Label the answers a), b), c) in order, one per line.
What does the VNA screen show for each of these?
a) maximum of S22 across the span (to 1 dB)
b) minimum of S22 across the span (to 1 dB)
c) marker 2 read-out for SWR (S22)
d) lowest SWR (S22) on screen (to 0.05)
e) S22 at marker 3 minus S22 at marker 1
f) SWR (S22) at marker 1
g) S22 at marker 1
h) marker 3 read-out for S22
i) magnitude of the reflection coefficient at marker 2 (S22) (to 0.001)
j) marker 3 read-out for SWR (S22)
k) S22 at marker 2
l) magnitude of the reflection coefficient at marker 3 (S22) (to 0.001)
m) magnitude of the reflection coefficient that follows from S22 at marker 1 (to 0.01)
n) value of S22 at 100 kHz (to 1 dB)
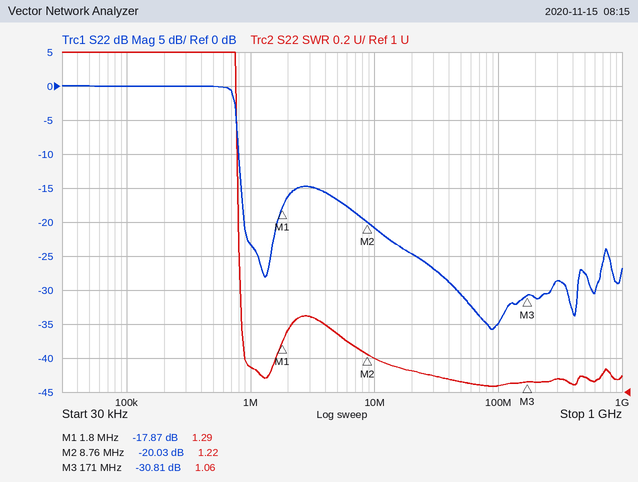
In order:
a) 0 dB
b) -36 dB
c) 1.22
d) 1.05
e) -12.94 dB
f) 1.29
g) -17.87 dB
h) -30.81 dB
i) 0.100
j) 1.06
k) -20.03 dB
l) 0.029
m) 0.13
n) 0 dB
